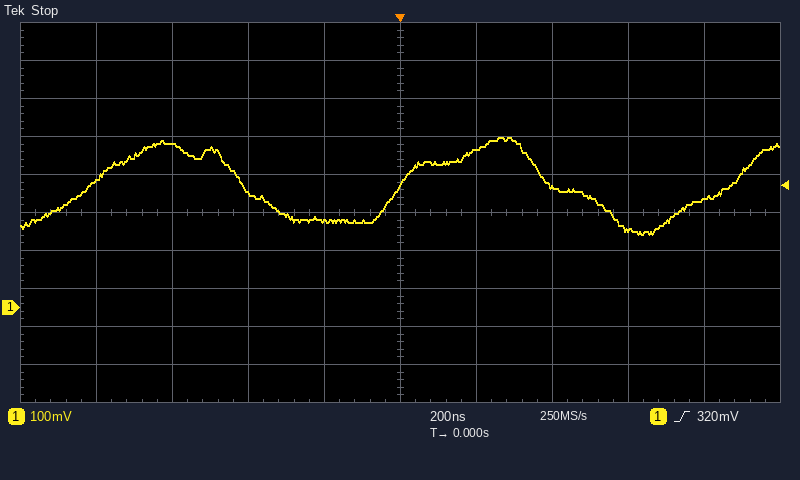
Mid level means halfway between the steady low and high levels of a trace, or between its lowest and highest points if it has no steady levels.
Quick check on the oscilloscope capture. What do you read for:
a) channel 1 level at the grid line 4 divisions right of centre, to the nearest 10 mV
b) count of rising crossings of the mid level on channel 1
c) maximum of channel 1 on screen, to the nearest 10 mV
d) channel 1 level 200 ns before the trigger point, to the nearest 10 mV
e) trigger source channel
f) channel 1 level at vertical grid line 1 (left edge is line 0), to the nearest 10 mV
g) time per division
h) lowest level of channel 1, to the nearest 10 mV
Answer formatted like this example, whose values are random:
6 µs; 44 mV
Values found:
290 mV; 3; 450 mV; 230 mV; channel 1; 340 mV; 200 ns; 190 mV
